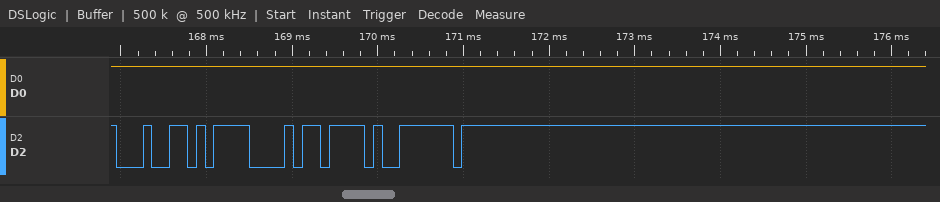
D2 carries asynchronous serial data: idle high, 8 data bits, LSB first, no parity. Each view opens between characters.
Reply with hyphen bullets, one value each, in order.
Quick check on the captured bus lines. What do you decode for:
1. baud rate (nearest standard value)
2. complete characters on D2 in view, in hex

- 9600 baud
- 64, 0F, 7B, 7E
